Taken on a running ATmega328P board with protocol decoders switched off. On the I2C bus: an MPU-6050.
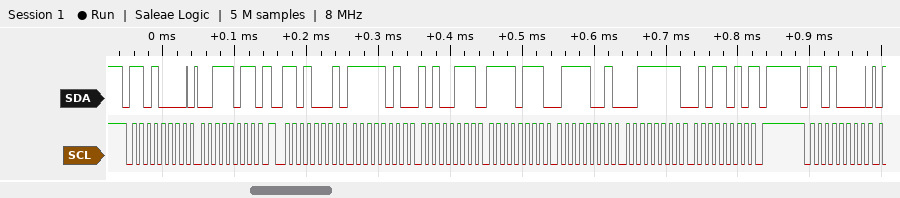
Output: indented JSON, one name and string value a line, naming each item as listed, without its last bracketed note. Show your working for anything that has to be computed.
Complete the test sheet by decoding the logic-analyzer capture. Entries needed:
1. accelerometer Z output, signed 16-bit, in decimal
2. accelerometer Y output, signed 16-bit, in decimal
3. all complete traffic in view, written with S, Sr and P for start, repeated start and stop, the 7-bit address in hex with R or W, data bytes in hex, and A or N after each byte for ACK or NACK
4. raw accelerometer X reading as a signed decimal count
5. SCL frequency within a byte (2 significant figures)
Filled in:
{
  "accelerometer Z output, signed 16-bit, in decimal": "0x3F5A = 16218",
  "accelerometer Y output, signed 16-bit, in decimal": "0xF779 = -2183",
  "all complete traffic in view, written with S, Sr and P for start, repeated start and stop, the 7-bit address in hex with R or W, data bytes in hex, and A or N after each byte for ACK or NACK": "S 68W A 3B A Sr 68R A FA A A7 A F7 A 79 A 3F A 5A N P S 68W A",
  "raw accelerometer X reading as a signed decimal count": "0xFAA7 = -1369",
  "SCL frequency within a byte": "100 kHz"
}
